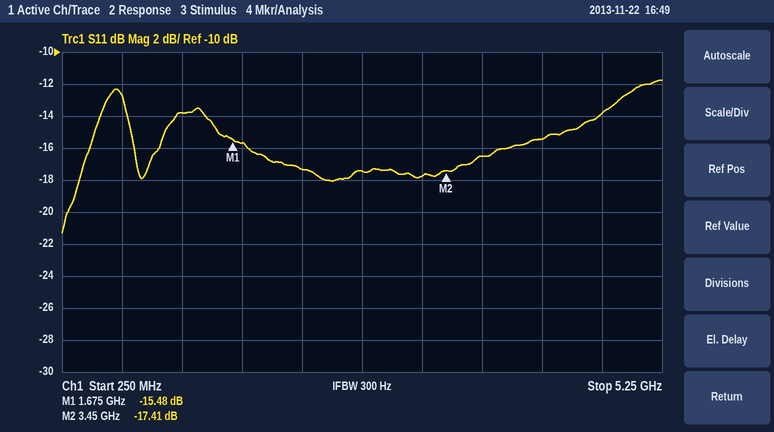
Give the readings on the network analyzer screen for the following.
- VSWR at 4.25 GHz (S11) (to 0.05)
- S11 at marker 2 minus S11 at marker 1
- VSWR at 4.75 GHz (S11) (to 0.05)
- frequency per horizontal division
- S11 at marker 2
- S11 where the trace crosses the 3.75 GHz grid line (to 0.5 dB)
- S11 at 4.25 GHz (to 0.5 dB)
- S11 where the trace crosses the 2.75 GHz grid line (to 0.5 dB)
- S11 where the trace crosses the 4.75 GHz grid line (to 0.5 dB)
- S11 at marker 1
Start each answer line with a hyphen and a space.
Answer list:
- 1.40
- -1.93 dB
- 1.50
- 500 MHz
- -17.41 dB
- -16.5 dB
- -15.5 dB
- -17.5 dB
- -14.0 dB
- -15.48 dB
